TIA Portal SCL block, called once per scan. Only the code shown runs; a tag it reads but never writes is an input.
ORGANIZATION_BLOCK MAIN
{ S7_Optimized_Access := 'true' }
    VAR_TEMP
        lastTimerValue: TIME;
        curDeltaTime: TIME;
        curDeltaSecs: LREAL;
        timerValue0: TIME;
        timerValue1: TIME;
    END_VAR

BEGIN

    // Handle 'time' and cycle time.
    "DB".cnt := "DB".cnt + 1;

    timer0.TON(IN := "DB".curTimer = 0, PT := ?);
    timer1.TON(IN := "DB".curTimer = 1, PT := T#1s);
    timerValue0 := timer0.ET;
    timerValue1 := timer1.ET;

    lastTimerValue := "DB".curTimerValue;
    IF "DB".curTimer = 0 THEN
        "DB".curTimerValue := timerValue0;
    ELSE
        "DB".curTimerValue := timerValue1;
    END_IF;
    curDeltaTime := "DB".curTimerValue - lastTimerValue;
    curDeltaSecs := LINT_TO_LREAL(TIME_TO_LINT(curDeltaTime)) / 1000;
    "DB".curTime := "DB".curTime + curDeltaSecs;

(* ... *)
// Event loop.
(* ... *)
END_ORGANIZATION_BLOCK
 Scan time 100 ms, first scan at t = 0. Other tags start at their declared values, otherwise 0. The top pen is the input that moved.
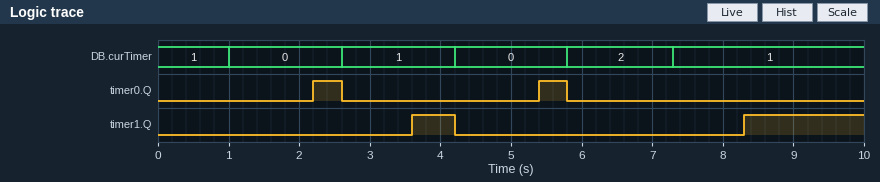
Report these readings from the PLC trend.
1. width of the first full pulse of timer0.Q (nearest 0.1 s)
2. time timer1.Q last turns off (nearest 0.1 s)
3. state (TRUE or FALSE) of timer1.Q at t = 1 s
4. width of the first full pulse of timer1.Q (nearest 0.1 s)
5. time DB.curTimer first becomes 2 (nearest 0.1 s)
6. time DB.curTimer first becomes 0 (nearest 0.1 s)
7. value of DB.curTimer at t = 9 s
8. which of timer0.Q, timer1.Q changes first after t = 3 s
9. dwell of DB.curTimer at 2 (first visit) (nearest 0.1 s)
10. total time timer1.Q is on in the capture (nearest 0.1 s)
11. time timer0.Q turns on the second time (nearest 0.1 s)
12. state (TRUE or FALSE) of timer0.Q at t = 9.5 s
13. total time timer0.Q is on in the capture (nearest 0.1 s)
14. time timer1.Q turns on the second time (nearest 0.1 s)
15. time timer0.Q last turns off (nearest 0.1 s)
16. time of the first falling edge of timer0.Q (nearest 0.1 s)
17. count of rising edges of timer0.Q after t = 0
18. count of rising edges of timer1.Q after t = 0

0.4 s
4.2 s
FALSE
0.6 s
5.8 s
1.0 s
1
timer1.Q
1.5 s
2.3 s
5.4 s
FALSE
0.8 s
8.3 s
5.8 s
2.6 s
2
2
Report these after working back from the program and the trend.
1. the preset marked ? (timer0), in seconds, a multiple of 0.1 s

1.2 s
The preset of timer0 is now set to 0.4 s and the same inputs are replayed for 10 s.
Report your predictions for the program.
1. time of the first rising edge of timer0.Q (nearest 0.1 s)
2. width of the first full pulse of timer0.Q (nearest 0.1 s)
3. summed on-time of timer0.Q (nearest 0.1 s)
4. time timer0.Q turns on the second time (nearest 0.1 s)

1.4 s
1.2 s
2.4 s
4.6 s
